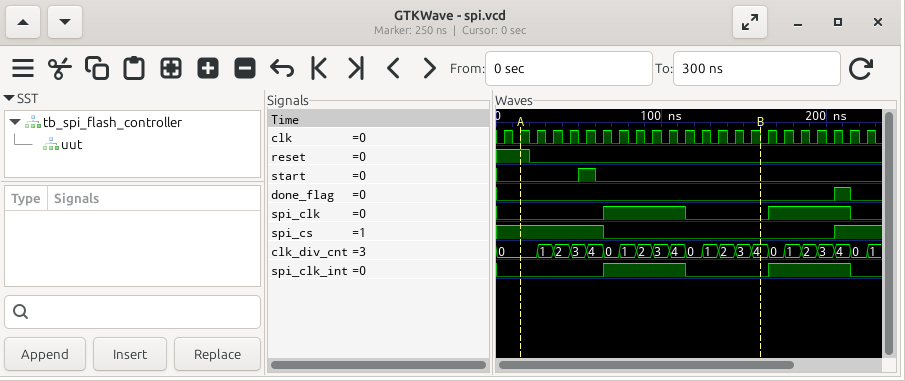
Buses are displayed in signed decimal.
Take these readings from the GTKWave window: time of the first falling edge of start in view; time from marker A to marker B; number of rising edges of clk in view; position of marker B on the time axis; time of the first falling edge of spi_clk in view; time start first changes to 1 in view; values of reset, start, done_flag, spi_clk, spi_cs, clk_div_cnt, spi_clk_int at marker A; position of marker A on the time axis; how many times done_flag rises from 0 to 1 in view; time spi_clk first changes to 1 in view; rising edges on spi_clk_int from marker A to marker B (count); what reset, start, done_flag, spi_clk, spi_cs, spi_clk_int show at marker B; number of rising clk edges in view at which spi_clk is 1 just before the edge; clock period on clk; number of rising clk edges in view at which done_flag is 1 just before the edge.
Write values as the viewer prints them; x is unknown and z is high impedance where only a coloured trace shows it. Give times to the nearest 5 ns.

60 ns
145 ns
23
160 ns
115 ns
50 ns
reset=1, start=0, done_flag=0, spi_clk=0, spi_cs=1, clk_div_cnt=0, spi_clk_int=0
15 ns
1
65 ns
1
reset=0, start=0, done_flag=0, spi_clk=0, spi_cs=0, spi_clk_int=0
10
10 ns
1
